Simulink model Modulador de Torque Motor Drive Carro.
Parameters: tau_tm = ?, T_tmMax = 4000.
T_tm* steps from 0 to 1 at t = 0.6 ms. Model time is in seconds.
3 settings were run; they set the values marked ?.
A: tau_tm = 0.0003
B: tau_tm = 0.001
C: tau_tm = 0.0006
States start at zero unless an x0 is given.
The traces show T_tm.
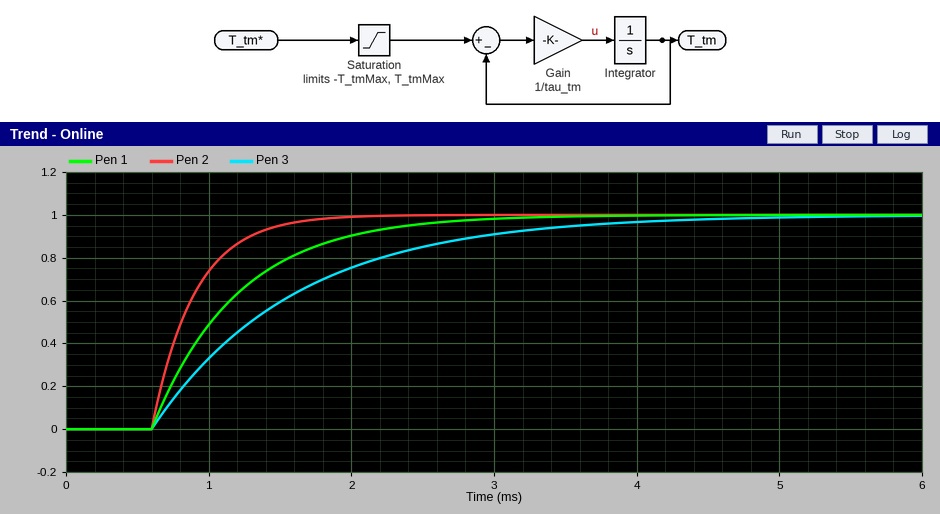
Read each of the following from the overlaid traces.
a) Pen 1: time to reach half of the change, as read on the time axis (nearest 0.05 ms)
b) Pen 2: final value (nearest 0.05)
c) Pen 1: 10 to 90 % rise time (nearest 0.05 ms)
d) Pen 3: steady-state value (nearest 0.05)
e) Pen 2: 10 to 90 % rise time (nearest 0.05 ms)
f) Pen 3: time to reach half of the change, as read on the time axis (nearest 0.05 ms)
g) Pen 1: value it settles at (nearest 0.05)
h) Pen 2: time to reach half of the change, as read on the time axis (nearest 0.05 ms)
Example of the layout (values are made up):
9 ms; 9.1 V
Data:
1.00 ms; 1.00; 1.30 ms; 1.00; 0.65 ms; 1.30 ms; 1.00; 0.80 ms
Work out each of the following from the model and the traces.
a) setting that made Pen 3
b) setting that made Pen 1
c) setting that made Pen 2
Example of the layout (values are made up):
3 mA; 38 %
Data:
B; C; A
